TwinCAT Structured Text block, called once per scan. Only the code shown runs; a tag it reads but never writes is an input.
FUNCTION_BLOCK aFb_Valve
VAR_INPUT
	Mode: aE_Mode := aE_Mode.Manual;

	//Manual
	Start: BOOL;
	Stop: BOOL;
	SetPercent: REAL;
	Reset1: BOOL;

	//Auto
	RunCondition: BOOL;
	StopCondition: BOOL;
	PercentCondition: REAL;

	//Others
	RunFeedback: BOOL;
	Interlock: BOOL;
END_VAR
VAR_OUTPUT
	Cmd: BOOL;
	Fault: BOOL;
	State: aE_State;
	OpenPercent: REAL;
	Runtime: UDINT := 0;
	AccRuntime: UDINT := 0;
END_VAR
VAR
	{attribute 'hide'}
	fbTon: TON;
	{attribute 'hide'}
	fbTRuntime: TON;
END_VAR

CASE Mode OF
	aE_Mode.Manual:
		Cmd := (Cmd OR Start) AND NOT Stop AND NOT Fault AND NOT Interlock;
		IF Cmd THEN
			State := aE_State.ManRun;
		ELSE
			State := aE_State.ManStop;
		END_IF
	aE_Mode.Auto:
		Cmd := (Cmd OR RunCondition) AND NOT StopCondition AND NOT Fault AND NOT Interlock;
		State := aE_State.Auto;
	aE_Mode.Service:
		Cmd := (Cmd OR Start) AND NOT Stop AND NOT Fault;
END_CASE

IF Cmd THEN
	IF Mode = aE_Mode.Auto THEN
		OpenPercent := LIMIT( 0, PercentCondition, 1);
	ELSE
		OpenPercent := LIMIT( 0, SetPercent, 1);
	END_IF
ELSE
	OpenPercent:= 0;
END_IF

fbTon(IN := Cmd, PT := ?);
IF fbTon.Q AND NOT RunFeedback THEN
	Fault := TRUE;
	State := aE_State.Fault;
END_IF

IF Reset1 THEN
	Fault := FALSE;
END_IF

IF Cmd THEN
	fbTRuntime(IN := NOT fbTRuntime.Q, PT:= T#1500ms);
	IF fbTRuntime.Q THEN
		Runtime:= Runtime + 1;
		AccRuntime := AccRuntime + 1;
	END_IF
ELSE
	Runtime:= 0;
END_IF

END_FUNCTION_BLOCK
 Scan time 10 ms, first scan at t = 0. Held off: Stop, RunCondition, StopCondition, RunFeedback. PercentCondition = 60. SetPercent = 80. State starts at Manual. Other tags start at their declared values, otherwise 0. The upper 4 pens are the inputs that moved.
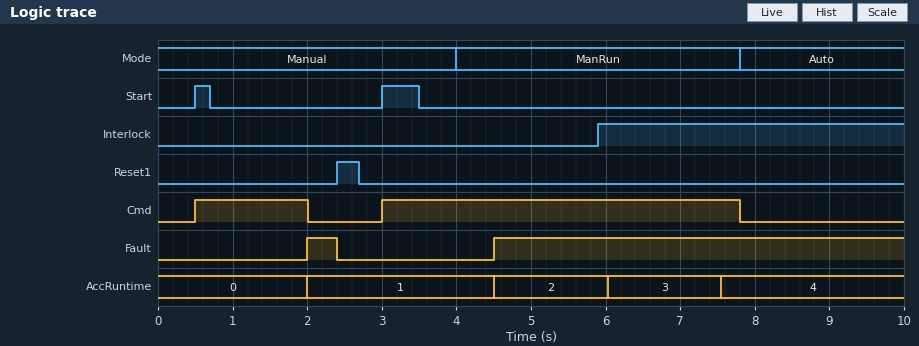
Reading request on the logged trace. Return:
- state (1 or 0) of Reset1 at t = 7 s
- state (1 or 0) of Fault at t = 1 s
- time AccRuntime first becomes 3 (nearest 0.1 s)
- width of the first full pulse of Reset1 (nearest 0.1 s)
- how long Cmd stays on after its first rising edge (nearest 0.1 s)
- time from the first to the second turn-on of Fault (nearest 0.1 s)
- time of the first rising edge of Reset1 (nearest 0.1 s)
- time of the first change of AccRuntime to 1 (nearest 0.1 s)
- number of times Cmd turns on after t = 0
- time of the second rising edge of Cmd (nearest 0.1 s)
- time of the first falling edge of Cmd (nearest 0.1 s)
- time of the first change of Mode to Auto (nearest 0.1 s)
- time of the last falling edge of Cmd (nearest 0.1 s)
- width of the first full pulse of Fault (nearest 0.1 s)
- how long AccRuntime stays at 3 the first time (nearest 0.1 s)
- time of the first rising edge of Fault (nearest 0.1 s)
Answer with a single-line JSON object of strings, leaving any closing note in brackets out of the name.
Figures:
{"state (1 or 0) of Reset1 at t = 7 s": "0", "state (1 or 0) of Fault at t = 1 s": "0", "time AccRuntime first becomes 3": "6.0 s", "width of the first full pulse of Reset1": "0.3 s", "how long Cmd stays on after its first rising edge": "1.5 s", "time from the first to the second turn-on of Fault": "2.5 s", "time of the first rising edge of Reset1": "2.4 s", "time of the first change of AccRuntime to 1": "2.0 s", "number of times Cmd turns on after t = 0": "2", "time of the second rising edge of Cmd": "3.0 s", "time of the first falling edge of Cmd": "2.0 s", "time of the first change of Mode to Auto": "7.8 s", "time of the last falling edge of Cmd": "7.8 s", "width of the first full pulse of Fault": "0.4 s", "how long AccRuntime stays at 3 the first time": "1.5 s", "time of the first rising edge of Fault": "2.0 s"}
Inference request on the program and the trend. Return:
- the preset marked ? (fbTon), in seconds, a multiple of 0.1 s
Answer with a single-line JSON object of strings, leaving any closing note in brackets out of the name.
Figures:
{"the preset marked ? (fbTon), in seconds, a multiple of 0.1 s": "1.5 s"}
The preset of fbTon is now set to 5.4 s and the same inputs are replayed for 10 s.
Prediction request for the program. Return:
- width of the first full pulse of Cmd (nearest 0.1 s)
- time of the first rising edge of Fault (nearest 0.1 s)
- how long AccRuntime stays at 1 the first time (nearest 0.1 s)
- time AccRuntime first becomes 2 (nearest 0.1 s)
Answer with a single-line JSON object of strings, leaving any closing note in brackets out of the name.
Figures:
{"width of the first full pulse of Cmd": "7.3 s", "time of the first rising edge of Fault": "5.9 s", "how long AccRuntime stays at 1 the first time": "1.5 s", "time AccRuntime first becomes 2": "3.5 s"}
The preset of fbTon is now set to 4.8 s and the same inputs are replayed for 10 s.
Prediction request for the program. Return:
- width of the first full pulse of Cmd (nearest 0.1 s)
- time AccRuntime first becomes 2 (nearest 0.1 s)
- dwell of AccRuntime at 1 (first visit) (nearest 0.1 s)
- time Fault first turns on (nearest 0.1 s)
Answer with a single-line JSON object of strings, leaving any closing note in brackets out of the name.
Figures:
{"width of the first full pulse of Cmd": "7.3 s", "time AccRuntime first becomes 2": "3.5 s", "dwell of AccRuntime at 1 (first visit)": "1.5 s", "time Fault first turns on": "5.3 s"}
